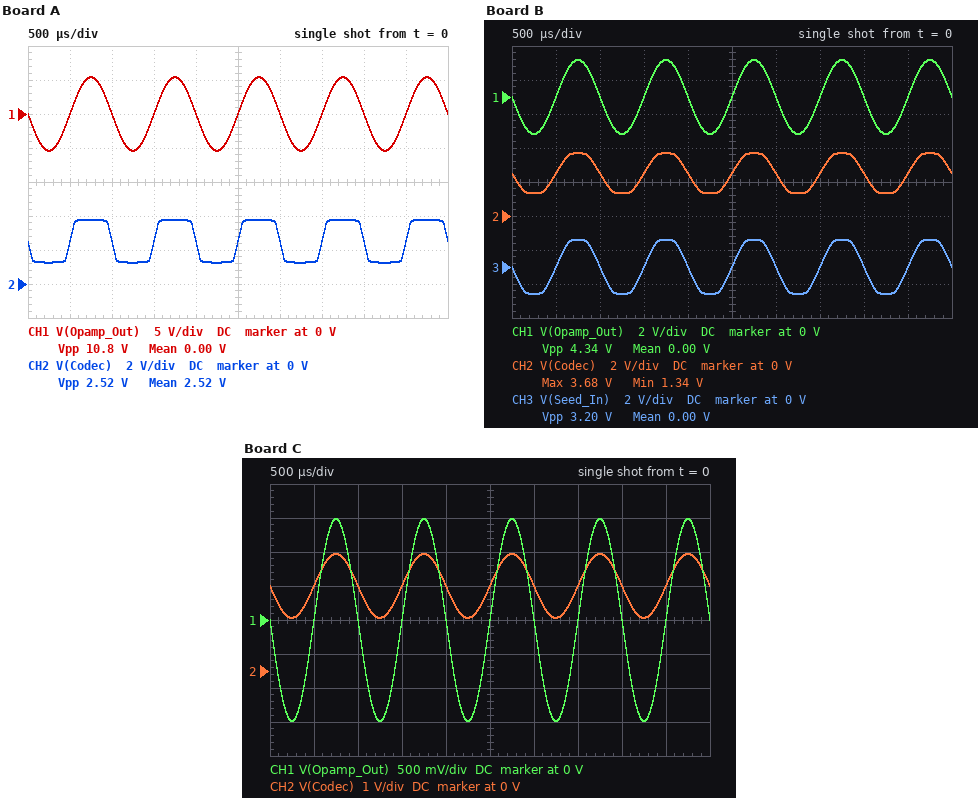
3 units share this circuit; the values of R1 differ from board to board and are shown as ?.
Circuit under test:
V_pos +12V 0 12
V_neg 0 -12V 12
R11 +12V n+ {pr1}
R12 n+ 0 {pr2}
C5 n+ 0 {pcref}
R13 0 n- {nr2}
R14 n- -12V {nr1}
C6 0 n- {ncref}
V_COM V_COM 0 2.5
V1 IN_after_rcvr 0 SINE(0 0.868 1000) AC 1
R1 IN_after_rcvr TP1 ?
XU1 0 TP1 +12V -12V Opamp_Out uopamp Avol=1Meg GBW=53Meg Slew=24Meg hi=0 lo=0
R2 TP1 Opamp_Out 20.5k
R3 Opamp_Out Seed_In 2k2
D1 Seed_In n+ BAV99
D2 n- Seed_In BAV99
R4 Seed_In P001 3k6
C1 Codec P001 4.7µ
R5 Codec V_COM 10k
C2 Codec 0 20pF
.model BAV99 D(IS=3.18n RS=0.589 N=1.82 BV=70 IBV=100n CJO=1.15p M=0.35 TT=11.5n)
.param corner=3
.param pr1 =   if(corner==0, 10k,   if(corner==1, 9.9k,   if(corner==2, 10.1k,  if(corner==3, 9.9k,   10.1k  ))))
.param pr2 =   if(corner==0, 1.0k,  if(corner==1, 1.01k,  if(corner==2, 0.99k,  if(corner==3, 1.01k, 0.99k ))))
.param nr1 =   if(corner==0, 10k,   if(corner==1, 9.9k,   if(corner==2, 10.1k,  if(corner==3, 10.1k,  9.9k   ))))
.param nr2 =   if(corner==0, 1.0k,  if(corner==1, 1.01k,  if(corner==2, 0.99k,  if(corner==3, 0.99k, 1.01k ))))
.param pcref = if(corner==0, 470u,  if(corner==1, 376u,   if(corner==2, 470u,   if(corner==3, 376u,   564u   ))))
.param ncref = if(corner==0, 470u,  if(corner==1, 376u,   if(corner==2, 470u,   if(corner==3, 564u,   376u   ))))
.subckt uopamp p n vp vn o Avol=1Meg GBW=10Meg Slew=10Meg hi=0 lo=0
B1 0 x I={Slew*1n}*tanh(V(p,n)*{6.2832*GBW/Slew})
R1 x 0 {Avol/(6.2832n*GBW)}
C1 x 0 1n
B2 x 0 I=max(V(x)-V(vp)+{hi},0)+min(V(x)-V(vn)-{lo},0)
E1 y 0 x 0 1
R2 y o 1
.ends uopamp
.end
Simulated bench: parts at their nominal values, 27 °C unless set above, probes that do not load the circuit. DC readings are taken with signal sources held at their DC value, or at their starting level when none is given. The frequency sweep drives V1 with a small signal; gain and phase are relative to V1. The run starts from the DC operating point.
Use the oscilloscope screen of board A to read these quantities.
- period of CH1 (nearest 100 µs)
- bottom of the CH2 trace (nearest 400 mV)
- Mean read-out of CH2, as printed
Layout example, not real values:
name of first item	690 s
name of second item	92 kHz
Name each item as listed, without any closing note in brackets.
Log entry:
period of CH1	1.0 ms
bottom of the CH2 trace	1.2 V
Mean read-out of CH2, as printed	2.52 V
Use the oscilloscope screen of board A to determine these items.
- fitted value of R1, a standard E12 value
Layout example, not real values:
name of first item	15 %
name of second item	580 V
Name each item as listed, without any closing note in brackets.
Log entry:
fitted value of R1, a standard E12 value	3.3 kΩ
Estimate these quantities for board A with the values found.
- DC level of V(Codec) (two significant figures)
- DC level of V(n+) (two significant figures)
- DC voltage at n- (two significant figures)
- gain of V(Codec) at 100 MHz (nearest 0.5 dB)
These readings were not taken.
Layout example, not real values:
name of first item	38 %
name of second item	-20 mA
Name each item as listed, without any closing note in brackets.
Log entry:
DC level of V(Codec)	2.5 V
DC level of V(n+)	1.1 V
DC voltage at n-	-1.1 V
gain of V(Codec) at 100 MHz	-49.5 dB
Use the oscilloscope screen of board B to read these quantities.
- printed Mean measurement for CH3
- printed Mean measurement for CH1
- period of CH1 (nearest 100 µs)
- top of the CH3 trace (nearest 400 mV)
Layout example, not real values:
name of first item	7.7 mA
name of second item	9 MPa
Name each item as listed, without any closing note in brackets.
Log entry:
printed Mean measurement for CH3	0.00 V
printed Mean measurement for CH1	0.00 V
period of CH1	1.0 ms
top of the CH3 trace	1.6 V
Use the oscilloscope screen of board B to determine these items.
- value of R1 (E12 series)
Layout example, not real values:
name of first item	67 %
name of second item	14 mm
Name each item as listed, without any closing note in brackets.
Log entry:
value of R1	8.2 kΩ
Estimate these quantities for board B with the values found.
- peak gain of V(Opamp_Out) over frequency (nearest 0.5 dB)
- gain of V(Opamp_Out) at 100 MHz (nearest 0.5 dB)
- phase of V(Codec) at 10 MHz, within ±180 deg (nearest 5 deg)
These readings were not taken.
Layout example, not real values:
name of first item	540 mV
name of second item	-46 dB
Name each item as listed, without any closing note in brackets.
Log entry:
peak gain of V(Opamp_Out) over frequency	8.0 dB
gain of V(Opamp_Out) at 100 MHz	-8.5 dB
phase of V(Codec) at 10 MHz, within ±180 deg	60 deg
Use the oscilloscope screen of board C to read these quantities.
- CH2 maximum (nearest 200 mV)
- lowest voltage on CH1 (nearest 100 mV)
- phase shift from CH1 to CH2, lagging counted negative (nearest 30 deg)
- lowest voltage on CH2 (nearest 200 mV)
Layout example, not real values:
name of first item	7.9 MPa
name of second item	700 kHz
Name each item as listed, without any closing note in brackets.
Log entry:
CH2 maximum	3.4 V
lowest voltage on CH1	-1.5 V
phase shift from CH1 to CH2, lagging counted negative	0 deg
lowest voltage on CH2	1.6 V
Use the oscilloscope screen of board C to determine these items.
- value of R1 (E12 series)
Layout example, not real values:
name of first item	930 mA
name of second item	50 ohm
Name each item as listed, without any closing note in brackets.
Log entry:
value of R1	12 kΩ
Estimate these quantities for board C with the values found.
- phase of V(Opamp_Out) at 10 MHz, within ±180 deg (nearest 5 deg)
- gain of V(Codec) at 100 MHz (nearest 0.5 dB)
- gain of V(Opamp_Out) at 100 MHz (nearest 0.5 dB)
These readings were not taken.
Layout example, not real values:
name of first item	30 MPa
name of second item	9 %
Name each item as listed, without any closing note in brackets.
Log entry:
phase of V(Opamp_Out) at 10 MHz, within ±180 deg	155 deg
gain of V(Codec) at 100 MHz	-52.0 dB
gain of V(Opamp_Out) at 100 MHz	-9.5 dB
